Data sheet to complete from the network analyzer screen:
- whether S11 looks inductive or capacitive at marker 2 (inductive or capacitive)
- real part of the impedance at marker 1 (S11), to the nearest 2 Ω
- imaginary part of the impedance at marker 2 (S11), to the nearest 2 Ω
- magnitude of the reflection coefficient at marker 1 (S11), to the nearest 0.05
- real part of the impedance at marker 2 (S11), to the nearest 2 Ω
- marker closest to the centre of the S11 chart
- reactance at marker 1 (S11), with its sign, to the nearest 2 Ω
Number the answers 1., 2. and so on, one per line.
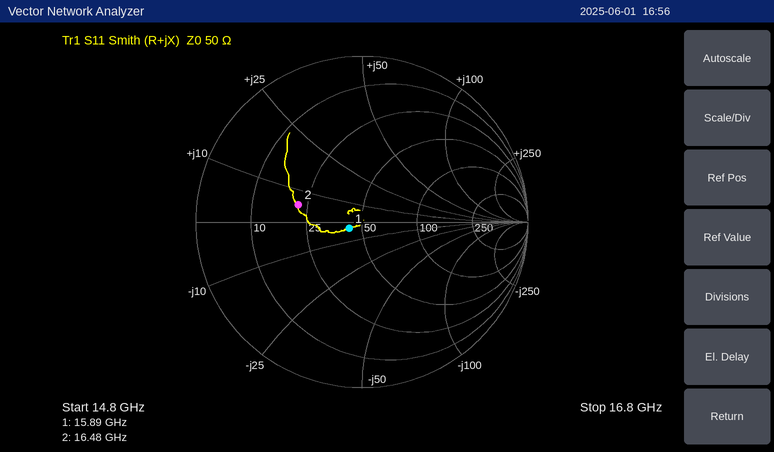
1. inductive
2. 42 Ω
3. +6 Ω
4. 0.10
5. 22 Ω
6. marker 1
7. -4 Ω
